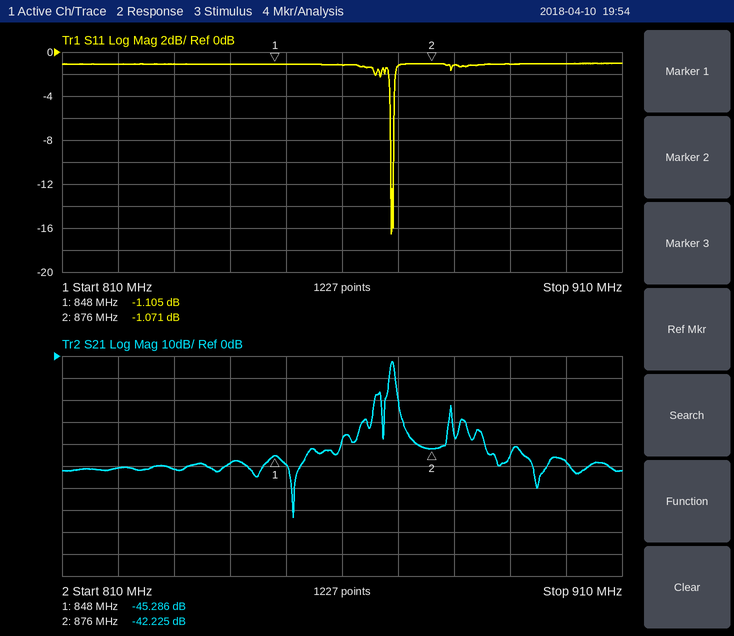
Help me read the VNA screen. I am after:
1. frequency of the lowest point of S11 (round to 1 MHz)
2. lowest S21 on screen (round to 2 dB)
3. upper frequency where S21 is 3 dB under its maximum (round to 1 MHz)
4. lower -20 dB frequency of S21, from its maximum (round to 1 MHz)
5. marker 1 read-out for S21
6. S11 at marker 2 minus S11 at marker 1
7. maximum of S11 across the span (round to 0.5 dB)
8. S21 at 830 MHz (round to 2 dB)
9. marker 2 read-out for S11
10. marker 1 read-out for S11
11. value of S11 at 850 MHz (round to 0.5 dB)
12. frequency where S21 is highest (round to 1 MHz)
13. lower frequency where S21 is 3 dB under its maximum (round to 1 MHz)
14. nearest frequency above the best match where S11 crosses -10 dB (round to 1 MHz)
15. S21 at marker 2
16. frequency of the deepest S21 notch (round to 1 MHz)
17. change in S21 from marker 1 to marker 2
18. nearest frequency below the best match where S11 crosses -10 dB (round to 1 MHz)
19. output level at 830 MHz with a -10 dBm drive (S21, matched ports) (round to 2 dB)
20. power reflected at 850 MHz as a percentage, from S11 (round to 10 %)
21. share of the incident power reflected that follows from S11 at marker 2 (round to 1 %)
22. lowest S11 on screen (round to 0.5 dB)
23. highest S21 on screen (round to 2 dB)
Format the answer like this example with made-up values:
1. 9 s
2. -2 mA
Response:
1. 869 MHz
2. -74 dB
3. 869 MHz
4. 868 MHz
5. -45.286 dB
6. 0.034 dB
7. -1.0 dB
8. -52 dB
9. -1.071 dB
10. -1.105 dB
11. -1.0 dB
12. 869 MHz
13. 869 MHz
14. 869 MHz
15. -42.225 dB
16. 851 MHz
17. 3.061 dB
18. 869 MHz
19. -62 dBm
20. 80 %
21. 78 %
22. -16.5 dB
23. -2 dB
